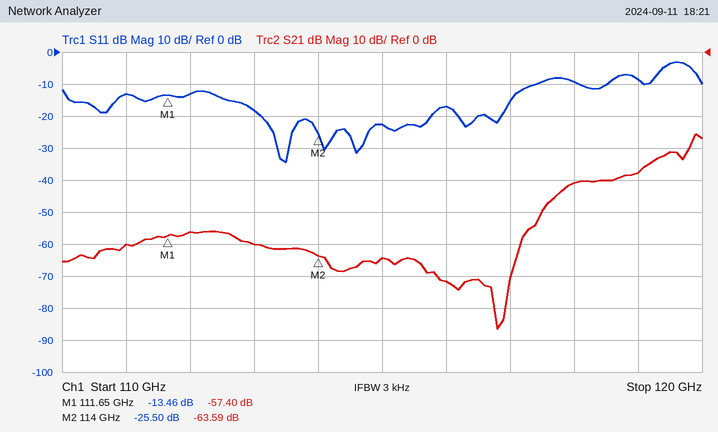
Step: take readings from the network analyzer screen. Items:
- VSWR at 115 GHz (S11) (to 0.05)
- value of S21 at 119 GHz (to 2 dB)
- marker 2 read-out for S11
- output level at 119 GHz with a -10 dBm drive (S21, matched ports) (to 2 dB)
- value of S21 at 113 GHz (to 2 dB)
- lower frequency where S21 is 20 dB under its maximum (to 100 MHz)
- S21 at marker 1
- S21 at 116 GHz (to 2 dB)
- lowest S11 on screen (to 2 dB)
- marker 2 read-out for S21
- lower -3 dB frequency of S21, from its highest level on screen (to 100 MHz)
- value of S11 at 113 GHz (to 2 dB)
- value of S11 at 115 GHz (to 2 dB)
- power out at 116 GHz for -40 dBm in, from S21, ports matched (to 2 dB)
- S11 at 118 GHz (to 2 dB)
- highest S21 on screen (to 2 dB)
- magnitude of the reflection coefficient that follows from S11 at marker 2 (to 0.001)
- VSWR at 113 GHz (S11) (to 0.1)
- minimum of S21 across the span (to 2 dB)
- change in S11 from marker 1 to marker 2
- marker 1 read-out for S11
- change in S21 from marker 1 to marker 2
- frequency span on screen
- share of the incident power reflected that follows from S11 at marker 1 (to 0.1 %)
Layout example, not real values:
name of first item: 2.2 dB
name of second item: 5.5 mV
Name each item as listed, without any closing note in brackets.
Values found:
VSWR at 115 GHz (S11): 1.15
value of S21 at 119 GHz: -38 dB
marker 2 read-out for S11: -25.50 dB
output level at 119 GHz with a -10 dBm drive (S21, matched ports): -48 dBm
value of S21 at 113 GHz: -60 dB
lower frequency where S21 is 20 dB under its maximum: 117.7 GHz
S21 at marker 1: -57.40 dB
S21 at 116 GHz: -72 dB
lowest S11 on screen: -34 dB
marker 2 read-out for S21: -63.59 dB
lower -3 dB frequency of S21, from its highest level on screen: 119.8 GHz
value of S11 at 113 GHz: -18 dB
value of S11 at 115 GHz: -22 dB
power out at 116 GHz for -40 dBm in, from S21, ports matched: -112 dBm
S11 at 118 GHz: -10 dB
highest S21 on screen: -26 dB
magnitude of the reflection coefficient that follows from S11 at marker 2: 0.053
VSWR at 113 GHz (S11): 1.3
minimum of S21 across the span: -86 dB
change in S11 from marker 1 to marker 2: -12.04 dB
marker 1 read-out for S11: -13.46 dB
change in S21 from marker 1 to marker 2: -6.19 dB
frequency span on screen: 10 GHz
share of the incident power reflected that follows from S11 at marker 1: 4.5 %
